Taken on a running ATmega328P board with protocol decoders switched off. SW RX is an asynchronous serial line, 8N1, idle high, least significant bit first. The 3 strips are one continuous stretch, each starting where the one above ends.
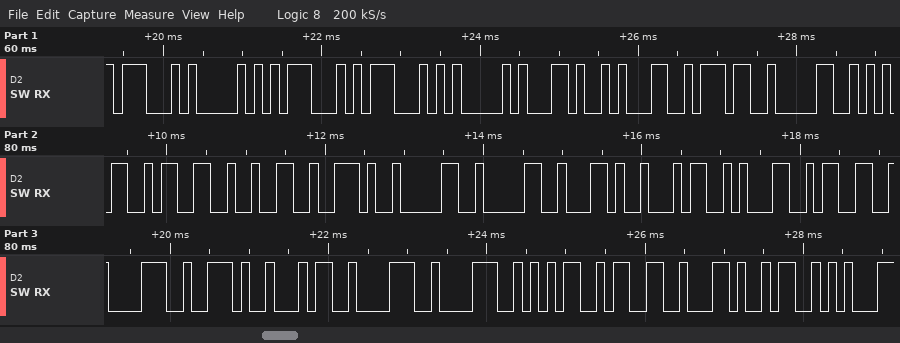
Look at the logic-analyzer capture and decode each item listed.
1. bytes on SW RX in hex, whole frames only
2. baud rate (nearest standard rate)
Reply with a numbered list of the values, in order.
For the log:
1. 47 50 47 47 41 2C 31 37 30 35 33 32 2E 30 30 2C 34 31 33 38 2E 34 38 38 35 33 2C 53
2. 9600 baud
